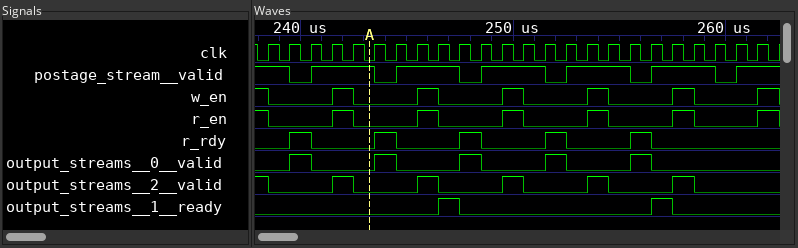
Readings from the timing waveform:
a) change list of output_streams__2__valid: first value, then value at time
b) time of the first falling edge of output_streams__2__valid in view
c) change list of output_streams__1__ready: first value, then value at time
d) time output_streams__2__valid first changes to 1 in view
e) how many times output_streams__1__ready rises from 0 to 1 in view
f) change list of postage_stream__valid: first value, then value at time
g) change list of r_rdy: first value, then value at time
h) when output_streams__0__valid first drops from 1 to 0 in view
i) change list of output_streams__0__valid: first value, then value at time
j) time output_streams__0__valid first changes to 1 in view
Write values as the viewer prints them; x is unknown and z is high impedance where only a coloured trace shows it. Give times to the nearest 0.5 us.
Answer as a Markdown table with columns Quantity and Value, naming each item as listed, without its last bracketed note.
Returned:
| Quantity | Value |
|---|---|
| change list of output_streams__2__valid: first value, then value at time | 1, 0 at 238.5 us, 1 at 241.5 us, 0 at 242.5 us, 1 at 245.5 us, 0 at 246.5 us, 1 at 249.5 us, 0 at 250.5 us, 1 at 253.5 us, 0 at 254.5 us, 1 at 257.5 us, 0 at 258.5 us |
| time of the first falling edge of output_streams__2__valid in view | 238.5 us |
| change list of output_streams__1__ready: first value, then value at time | 0, 1 at 246.5 us, 0 at 247.5 us, 1 at 256.5 us, 0 at 257.5 us |
| time output_streams__2__valid first changes to 1 in view | 241.5 us |
| how many times output_streams__1__ready rises from 0 to 1 in view | 2 |
| change list of postage_stream__valid: first value, then value at time | 1, 0 at 239.5 us, 1 at 240.5 us, 0 at 243.5 us, 1 at 244.5 us, 0 at 247.5 us, 1 at 248.5 us, 0 at 251.5 us, 1 at 252.5 us, 0 at 255.5 us, 1 at 256.5 us, 0 at 259.5 us, 1 at 260.5 us |
| change list of r_rdy: first value, then value at time | 0, 1 at 239.5 us, 0 at 240.5 us, 1 at 243.5 us, 0 at 244.5 us, 1 at 247.5 us, 0 at 248.5 us, 1 at 251.5 us, 0 at 252.5 us, 1 at 255.5 us, 0 at 256.5 us |
| when output_streams__0__valid first drops from 1 to 0 in view | 240.5 us |
| change list of output_streams__0__valid: first value, then value at time | 0, 1 at 239.5 us, 0 at 240.5 us, 1 at 243.5 us, 0 at 244.5 us, 1 at 247.5 us, 0 at 248.5 us, 1 at 251.5 us, 0 at 252.5 us, 1 at 255.5 us, 0 at 256.5 us |
| time output_streams__0__valid first changes to 1 in view | 239.5 us |
